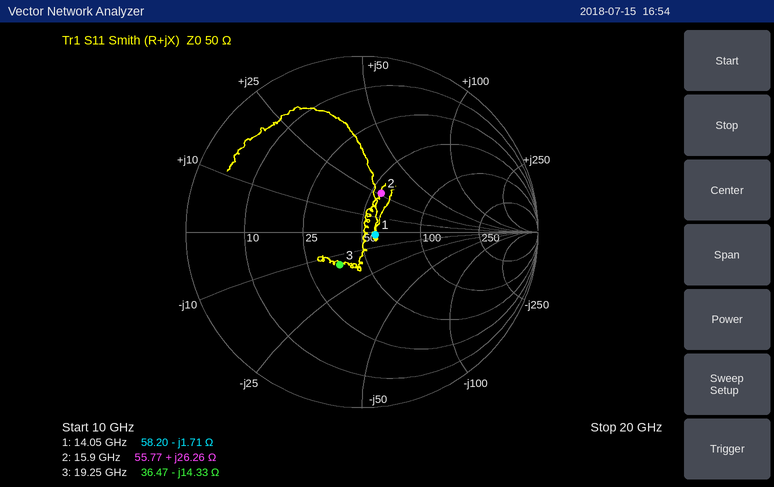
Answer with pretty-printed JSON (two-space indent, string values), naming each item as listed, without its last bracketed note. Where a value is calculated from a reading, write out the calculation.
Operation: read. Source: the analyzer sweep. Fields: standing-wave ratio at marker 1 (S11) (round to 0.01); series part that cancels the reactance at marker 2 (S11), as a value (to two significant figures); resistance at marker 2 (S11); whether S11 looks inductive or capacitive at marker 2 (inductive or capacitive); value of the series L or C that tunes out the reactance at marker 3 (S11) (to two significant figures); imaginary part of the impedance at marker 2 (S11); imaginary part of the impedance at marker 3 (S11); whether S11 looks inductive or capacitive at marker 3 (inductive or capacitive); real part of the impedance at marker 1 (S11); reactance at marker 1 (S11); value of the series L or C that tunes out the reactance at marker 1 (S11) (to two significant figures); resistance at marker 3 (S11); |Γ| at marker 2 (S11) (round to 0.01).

{
  "standing-wave ratio at marker 1 (S11)": "1.17",
  "series part that cancels the reactance at marker 2 (S11), as a value": "C = 1/(2π × 15.9 GHz × 26.26 Ω) ≈ 381 fF, so 380 fF to two significant figures",
  "resistance at marker 2": "55.77 Ω",
  "whether S11 looks inductive or capacitive at marker 2": "inductive",
  "value of the series L or C that tunes out the reactance at marker 3 (S11)": "L = 14.33 Ω/(2π × 19.25 GHz) ≈ 118 pH, so 120 pH to two significant figures",
  "imaginary part of the impedance at marker 2": "+26.26 Ω",
  "imaginary part of the impedance at marker 3": "-14.33 Ω",
  "whether S11 looks inductive or capacitive at marker 3": "capacitive",
  "real part of the impedance at marker 1": "58.20 Ω",
  "reactance at marker 1": "-1.71 Ω",
  "value of the series L or C that tunes out the reactance at marker 1 (S11)": "L = 1.71 Ω/(2π × 14.05 GHz) ≈ 19 pH",
  "resistance at marker 3": "36.47 Ω",
  "|Γ| at marker 2 (S11)": "0.25"
}
